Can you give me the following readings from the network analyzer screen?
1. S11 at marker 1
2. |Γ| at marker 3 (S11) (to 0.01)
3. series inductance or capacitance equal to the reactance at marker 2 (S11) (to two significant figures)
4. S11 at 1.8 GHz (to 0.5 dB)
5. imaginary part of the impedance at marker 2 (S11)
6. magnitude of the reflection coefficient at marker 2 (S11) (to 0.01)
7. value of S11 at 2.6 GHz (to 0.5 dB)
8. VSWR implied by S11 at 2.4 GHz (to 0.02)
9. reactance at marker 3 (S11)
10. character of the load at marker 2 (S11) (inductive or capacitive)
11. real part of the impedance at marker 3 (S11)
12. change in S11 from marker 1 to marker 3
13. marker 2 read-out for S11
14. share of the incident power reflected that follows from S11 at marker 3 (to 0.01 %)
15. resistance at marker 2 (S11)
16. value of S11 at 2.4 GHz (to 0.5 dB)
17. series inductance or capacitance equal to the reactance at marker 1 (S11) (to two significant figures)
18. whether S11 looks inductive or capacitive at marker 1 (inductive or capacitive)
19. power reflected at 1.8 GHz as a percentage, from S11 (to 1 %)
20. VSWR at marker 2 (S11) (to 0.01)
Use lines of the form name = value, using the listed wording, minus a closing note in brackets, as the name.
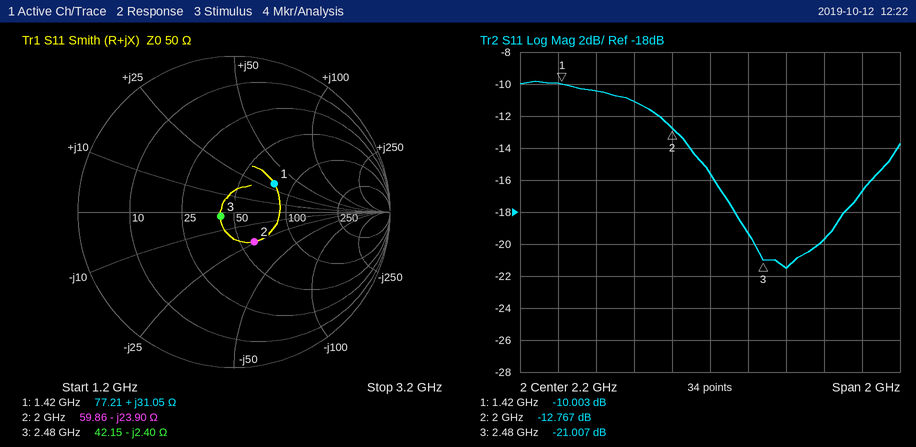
S11 at marker 1 = -10.003 dB
|Γ| at marker 3 (S11) = 0.09
series inductance or capacitance equal to the reactance at marker 2 (S11) = 3.3 pF
S11 at 1.8 GHz = -11.0 dB
imaginary part of the impedance at marker 2 = -23.90 Ω
magnitude of the reflection coefficient at marker 2 (S11) = 0.23
value of S11 at 2.6 GHz = -21.5 dB
VSWR implied by S11 at 2.4 GHz = 1.24
reactance at marker 3 = -2.40 Ω
character of the load at marker 2 (S11) = capacitive
real part of the impedance at marker 3 = 42.15 Ω
change in S11 from marker 1 to marker 3 = -11.004 dB
marker 2 read-out for S11 = -12.767 dB
share of the incident power reflected that follows from S11 at marker 3 = 0.79 %
resistance at marker 2 = 59.86 Ω
value of S11 at 2.4 GHz = -19.5 dB
series inductance or capacitance equal to the reactance at marker 1 (S11) = 3.5 nH
whether S11 looks inductive or capacitive at marker 1 = inductive
power reflected at 1.8 GHz as a percentage, from S11 = 8 %
VSWR at marker 2 (S11) = 1.60
